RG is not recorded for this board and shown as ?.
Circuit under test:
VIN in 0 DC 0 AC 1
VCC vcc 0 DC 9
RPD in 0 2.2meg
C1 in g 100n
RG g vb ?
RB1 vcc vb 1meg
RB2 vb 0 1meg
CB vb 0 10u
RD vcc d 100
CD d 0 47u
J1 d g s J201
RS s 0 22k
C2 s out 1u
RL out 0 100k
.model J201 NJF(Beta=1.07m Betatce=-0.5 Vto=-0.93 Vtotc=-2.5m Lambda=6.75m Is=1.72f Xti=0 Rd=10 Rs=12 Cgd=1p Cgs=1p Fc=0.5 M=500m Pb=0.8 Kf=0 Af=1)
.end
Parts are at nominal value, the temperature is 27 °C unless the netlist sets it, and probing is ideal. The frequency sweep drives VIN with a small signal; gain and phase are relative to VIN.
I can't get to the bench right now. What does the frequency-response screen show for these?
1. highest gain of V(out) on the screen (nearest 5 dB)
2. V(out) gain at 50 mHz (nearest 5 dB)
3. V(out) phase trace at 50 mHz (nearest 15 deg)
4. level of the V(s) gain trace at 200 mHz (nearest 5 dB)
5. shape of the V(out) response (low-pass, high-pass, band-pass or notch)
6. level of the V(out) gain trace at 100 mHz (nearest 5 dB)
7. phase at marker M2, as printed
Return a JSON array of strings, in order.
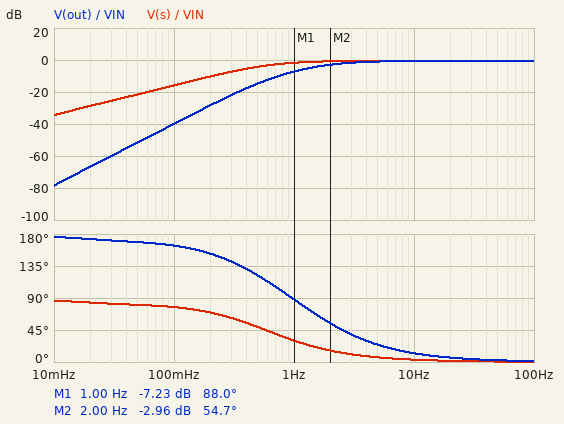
["0 dB", "-50 dB", "165 deg", "-10 dB", "high-pass", "-40 dB", "54.7 deg"]
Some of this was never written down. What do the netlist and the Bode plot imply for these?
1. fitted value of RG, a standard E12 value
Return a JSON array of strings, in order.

["2.7 MΩ"]
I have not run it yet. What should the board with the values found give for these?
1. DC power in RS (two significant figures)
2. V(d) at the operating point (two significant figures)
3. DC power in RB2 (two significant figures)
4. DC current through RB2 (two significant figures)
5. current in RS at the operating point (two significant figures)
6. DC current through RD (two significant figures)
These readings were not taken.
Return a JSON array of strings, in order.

["1.1 mW", "9.0 V", "20 µW", "4.5 µA", "230 µA", "230 µA"]
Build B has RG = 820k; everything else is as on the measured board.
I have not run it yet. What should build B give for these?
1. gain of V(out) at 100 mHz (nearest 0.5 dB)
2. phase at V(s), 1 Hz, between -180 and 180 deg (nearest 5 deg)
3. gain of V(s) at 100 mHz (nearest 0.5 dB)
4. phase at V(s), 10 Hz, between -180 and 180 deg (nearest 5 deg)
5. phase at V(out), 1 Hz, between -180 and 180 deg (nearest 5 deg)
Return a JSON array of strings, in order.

["-49.5 dB", "60 deg", "-25.5 dB", "10 deg", "120 deg"]
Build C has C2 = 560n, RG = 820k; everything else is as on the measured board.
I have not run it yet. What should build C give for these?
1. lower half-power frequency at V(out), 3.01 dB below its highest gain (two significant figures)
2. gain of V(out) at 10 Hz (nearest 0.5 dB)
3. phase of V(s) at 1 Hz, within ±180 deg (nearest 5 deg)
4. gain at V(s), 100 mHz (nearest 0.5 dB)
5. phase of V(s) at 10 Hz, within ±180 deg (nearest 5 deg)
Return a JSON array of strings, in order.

["3.7 Hz", "-1.0 dB", "60 deg", "-25.5 dB", "10 deg"]
